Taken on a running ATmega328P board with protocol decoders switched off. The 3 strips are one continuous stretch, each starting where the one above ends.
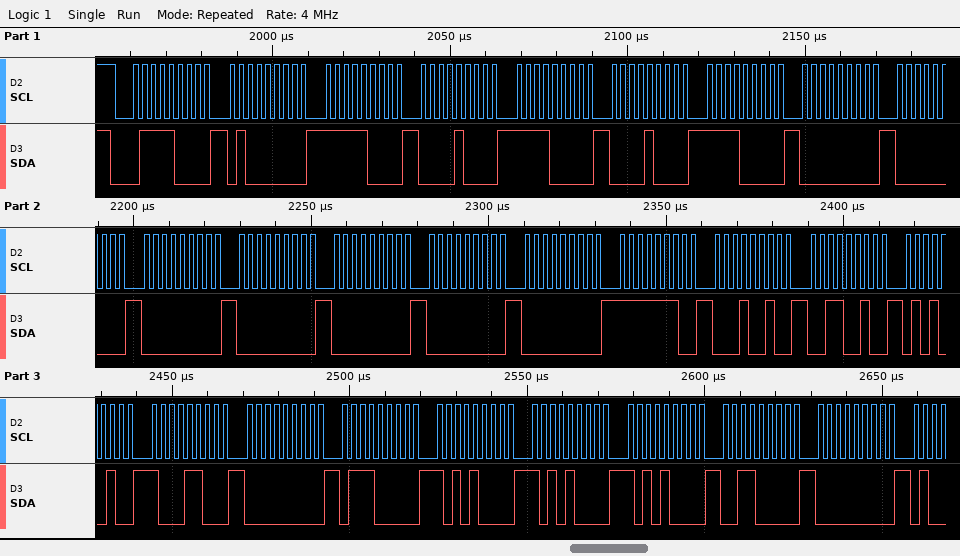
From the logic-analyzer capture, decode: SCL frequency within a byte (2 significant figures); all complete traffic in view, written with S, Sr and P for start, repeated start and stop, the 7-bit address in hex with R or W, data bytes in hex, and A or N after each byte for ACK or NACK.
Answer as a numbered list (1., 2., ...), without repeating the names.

1. 400 kHz
2. S 3CW A 40 A F8 A 08 A F0 A 08 A F0 A 00 A 00 A 00 A 00 A 00 A 00 A 00 A FE A 12 A 32 A 52 A 8C A 00 A 70 A A8 A A8 A A8 A 30 A 00 A
